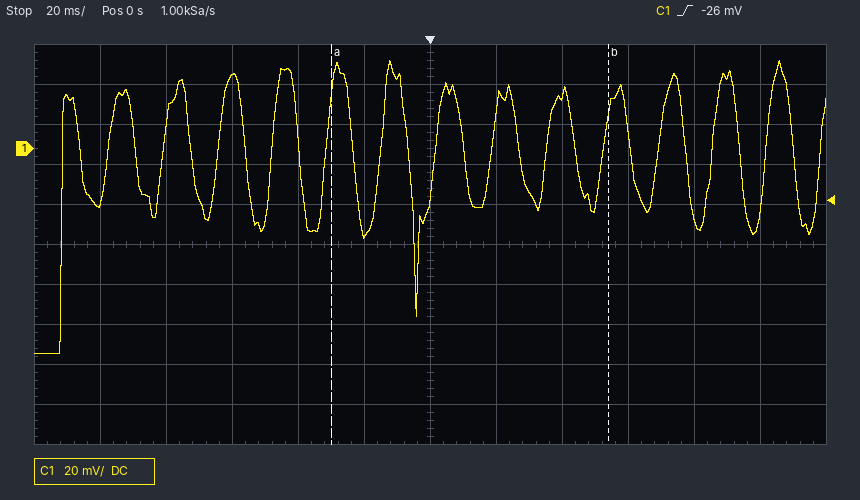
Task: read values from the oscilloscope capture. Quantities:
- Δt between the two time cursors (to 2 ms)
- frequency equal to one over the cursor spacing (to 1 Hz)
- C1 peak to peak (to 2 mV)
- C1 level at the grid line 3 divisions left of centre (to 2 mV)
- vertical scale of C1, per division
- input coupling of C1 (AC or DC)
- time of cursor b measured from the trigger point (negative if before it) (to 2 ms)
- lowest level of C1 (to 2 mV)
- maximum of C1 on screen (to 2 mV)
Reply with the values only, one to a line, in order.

84 ms
12 Hz
146 mV
36 mV
20 mV
DC
+54 ms
-102 mV
44 mV
